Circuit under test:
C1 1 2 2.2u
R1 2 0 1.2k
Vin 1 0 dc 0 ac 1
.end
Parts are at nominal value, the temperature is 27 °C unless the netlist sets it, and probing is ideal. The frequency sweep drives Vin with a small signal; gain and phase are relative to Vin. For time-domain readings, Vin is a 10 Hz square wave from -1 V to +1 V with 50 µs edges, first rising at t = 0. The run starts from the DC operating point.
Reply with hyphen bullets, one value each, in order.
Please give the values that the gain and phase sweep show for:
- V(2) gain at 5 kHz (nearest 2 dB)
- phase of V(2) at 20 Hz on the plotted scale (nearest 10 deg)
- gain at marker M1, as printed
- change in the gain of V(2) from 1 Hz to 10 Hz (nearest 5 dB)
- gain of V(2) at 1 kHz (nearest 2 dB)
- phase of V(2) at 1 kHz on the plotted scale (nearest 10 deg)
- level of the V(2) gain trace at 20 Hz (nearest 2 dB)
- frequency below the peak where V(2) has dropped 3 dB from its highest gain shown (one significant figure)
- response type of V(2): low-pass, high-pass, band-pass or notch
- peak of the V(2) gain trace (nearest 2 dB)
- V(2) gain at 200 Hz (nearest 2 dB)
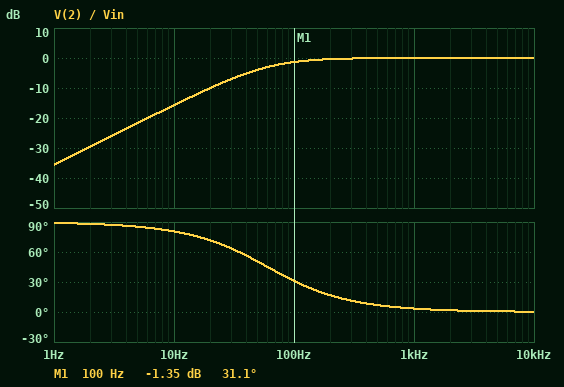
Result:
- 0 dB
- 70 deg
- -1.35 dB
- 20 dB
- 0 dB
- 0 deg
- -10 dB
- 60 Hz
- high-pass
- 0 dB
- 0 dB
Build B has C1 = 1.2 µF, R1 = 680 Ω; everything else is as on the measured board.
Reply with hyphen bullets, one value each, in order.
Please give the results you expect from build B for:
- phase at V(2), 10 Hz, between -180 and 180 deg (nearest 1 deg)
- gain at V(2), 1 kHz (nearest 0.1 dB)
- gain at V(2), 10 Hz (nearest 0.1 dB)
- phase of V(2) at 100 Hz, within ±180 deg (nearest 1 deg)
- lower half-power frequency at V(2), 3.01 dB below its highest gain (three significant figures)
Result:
- 87 deg
- -0.2 dB
- -25.8 dB
- 63 deg
- 195 Hz
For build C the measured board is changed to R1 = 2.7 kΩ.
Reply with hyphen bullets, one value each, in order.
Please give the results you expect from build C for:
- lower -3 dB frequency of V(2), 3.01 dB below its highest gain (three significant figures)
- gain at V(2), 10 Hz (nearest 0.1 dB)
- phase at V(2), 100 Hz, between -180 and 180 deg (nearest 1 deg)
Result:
- 26.8 Hz
- -9.1 dB
- 15 deg
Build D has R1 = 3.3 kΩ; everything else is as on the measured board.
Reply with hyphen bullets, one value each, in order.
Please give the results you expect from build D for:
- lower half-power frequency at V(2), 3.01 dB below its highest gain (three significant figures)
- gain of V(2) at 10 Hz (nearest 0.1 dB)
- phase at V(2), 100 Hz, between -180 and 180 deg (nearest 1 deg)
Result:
- 21.9 Hz
- -7.6 dB
- 12 deg
